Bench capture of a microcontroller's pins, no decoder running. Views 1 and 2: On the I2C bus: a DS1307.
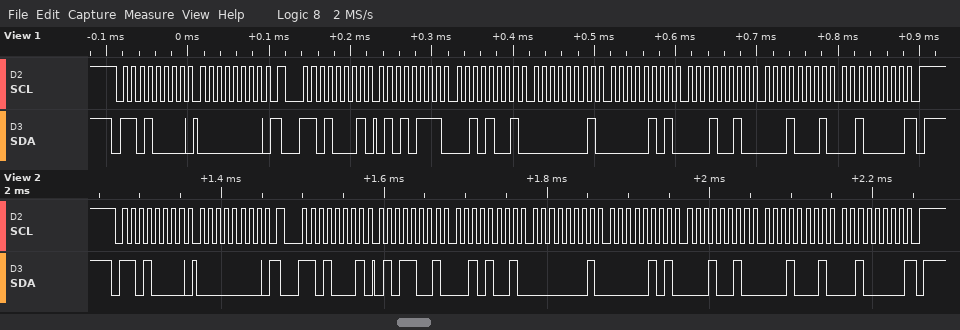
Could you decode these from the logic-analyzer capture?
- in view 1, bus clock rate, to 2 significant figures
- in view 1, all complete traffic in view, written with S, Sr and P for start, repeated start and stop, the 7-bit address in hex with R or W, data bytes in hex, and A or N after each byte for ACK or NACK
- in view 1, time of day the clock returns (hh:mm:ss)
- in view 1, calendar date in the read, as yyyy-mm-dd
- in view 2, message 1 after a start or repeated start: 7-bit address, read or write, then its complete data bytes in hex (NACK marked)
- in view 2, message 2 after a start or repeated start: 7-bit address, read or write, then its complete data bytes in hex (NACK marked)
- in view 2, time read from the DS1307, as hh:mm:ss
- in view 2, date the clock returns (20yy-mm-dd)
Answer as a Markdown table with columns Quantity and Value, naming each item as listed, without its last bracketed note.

| Quantity | Value |
|---|---|
| in view 1, bus clock rate, to 2 significant figures | 100 kHz |
| in view 1, all complete traffic in view, written with S, Sr and P for start, repeated start and stop, the 7-bit address in hex with R or W, data bytes in hex, and A or N after each byte for ACK or NACK | S 68W A 00 A Sr 68R A 57 A 29 A 01 A 05 A 12 A 11 A 20 N P |
| in view 1, time of day the clock returns | 01:29:57 |
| in view 1, calendar date in the read, as yyyy-mm-dd | 2020-11-12 |
| in view 2, message 1 after a start or repeated start: 7-bit address, read or write, then its complete data bytes in hex | 0x68 write: 00 |
| in view 2, message 2 after a start or repeated start: 7-bit address, read or write, then its complete data bytes in hex | 0x68 read: 59 29 01 05 12 11 20 NACK |
| in view 2, time read from the DS1307, as hh:mm:ss | 01:29:59 |
| in view 2, date the clock returns | 2020-11-12 |
